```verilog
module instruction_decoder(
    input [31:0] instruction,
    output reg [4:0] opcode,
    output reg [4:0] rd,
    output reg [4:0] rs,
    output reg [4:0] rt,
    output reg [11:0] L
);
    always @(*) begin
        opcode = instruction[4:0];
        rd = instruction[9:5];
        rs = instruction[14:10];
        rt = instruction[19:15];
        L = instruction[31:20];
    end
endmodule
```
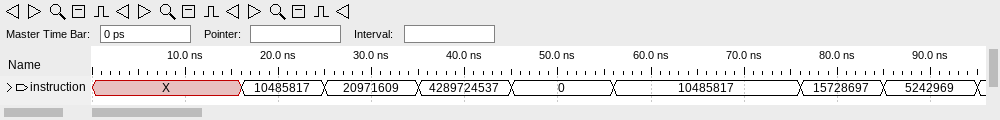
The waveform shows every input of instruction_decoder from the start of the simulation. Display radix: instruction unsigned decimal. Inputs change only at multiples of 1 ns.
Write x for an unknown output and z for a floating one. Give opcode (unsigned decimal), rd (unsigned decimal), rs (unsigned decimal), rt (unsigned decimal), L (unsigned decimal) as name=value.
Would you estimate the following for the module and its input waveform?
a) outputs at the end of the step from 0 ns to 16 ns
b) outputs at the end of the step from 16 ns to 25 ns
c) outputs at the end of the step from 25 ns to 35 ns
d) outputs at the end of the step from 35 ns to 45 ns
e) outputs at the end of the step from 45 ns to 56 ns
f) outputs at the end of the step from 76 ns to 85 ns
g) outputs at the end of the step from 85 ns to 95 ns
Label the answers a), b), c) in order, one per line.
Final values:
a) opcode=x, rd=x, rs=x, rt=x, L=x
b) opcode=25, rd=1, rs=0, rt=0, L=10
c) opcode=25, rd=2, rs=0, rt=0, L=20
d) opcode=25, rd=3, rs=0, rt=0, L=4091
e) opcode=0, rd=0, rs=0, rt=0, L=0
f) opcode=25, rd=1, rs=0, rt=0, L=15
g) opcode=25, rd=2, rs=0, rt=0, L=5
